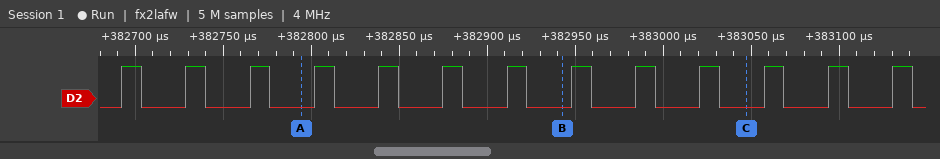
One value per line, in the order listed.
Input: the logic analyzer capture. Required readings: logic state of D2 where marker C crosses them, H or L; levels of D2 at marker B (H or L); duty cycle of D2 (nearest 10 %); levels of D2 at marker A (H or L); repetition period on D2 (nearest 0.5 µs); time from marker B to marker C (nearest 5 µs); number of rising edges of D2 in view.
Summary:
D2=L
D2=L
30 %
D2=L
36.5 µs
105 µs
13
